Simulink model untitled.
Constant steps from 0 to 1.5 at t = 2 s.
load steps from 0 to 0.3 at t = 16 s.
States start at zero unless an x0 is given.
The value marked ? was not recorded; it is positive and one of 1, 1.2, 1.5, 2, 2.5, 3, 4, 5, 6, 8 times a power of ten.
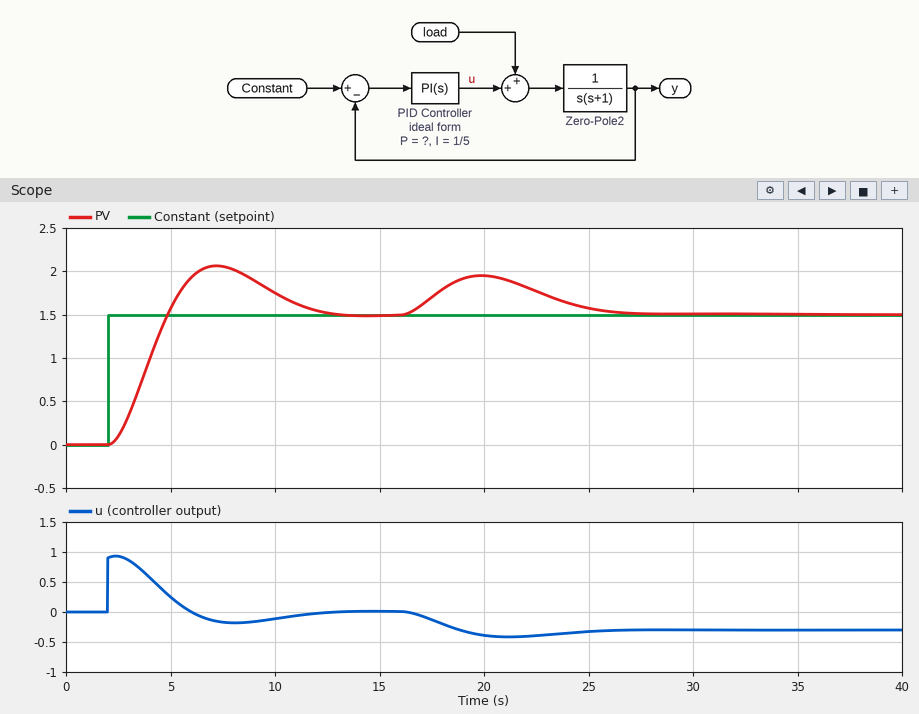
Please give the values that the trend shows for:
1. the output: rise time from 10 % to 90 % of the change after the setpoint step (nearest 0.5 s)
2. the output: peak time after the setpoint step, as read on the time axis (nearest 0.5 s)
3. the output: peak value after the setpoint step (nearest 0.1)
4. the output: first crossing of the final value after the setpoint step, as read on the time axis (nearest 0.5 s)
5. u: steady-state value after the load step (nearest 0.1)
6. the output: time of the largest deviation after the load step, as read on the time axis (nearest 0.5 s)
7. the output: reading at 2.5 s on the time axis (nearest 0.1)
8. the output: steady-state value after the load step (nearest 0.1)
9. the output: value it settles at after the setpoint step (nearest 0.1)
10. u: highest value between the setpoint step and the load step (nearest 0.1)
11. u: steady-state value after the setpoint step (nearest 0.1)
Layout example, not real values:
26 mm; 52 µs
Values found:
2.0 s; 7.0 s; 2.1; 5.0 s; -0.3; 20.0 s; 0.1; 1.5; 1.5; 0.9; 0.0
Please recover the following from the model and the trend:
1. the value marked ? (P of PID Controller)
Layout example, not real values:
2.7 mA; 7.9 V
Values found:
0.6
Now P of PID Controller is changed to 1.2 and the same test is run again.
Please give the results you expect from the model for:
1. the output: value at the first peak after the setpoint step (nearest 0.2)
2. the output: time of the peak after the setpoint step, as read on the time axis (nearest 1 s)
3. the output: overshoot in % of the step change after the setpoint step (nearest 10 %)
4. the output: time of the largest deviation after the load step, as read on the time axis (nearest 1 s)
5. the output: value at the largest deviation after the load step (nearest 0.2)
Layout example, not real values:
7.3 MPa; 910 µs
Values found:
2.2; 5 s; 40 %; 19 s; 1.8
